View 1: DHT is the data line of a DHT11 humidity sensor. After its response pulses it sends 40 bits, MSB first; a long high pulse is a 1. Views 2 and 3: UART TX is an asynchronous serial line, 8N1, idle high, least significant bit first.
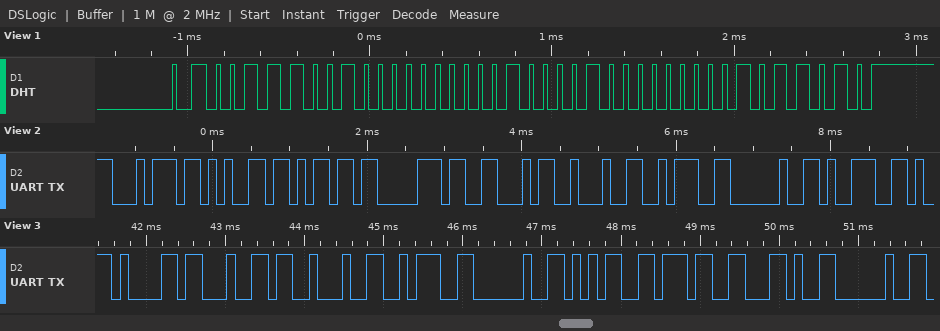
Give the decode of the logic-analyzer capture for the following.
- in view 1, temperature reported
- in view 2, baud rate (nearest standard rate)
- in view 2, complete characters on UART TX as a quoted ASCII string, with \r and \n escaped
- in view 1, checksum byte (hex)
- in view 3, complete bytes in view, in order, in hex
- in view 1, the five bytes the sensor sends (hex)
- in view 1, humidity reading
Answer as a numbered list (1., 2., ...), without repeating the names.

1. 33.0 °C
2. 9600 baud
3. "tempF\": 9"
4. 0x5A
5. 61 64 22 3A 20 35 37 2C 20
6. 39 00 21 00 5A
7. 57 %
